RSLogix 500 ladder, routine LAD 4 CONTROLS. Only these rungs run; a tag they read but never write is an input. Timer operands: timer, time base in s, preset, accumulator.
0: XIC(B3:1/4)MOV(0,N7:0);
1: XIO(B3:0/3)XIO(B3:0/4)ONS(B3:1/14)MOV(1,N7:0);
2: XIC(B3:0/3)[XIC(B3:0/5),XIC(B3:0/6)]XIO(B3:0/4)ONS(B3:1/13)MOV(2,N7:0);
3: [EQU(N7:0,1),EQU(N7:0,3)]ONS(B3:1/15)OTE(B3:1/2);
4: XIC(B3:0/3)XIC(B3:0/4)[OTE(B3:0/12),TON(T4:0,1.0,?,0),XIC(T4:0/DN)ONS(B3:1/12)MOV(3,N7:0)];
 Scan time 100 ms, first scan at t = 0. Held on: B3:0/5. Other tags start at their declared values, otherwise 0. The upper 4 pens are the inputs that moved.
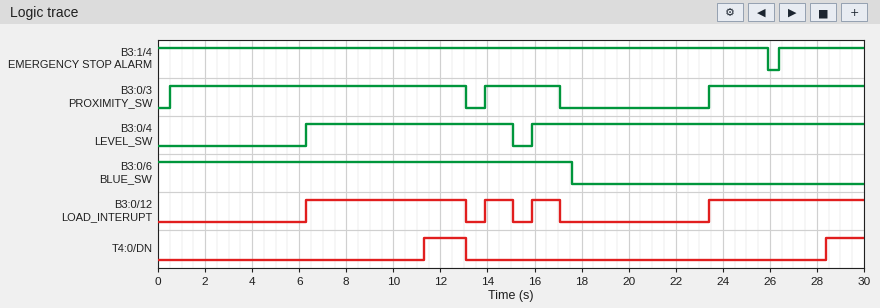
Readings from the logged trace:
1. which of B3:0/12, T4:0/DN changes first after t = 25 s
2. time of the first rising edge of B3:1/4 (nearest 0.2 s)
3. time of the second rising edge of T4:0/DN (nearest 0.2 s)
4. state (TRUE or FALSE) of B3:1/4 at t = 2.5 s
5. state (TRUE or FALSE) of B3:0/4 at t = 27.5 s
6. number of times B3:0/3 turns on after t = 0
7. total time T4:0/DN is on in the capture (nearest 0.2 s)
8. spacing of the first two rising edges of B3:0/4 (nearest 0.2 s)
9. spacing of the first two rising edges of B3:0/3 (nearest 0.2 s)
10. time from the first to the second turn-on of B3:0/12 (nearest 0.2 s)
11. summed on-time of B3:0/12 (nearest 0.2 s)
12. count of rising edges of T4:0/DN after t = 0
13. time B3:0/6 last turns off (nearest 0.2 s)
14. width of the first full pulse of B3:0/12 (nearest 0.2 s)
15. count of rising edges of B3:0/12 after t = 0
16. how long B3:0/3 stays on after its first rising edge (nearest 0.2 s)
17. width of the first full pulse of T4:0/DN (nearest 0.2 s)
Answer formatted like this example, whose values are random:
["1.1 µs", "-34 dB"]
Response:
["T4:0/DN", "26.4 s", "28.4 s", "TRUE", "TRUE", "3", "3.4 s", "9.6 s", "13.4 s", "7.6 s", "15.8 s", "2", "17.6 s", "6.8 s", "4", "12.6 s", "1.8 s"]
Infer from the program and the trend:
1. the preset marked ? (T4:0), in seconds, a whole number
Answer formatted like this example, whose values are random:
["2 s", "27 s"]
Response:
["5 s"]
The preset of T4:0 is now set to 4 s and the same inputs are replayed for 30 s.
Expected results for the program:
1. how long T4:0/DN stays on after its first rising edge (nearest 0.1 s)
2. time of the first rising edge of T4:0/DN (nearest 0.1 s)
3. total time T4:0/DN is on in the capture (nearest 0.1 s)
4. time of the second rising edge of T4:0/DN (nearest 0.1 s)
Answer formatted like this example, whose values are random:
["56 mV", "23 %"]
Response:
["2.8 s", "10.3 s", "5.4 s", "27.4 s"]
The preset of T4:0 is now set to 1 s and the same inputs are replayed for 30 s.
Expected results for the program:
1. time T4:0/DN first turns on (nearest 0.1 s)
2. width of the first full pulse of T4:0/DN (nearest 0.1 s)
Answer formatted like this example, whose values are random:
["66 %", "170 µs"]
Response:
["7.3 s", "5.8 s"]
